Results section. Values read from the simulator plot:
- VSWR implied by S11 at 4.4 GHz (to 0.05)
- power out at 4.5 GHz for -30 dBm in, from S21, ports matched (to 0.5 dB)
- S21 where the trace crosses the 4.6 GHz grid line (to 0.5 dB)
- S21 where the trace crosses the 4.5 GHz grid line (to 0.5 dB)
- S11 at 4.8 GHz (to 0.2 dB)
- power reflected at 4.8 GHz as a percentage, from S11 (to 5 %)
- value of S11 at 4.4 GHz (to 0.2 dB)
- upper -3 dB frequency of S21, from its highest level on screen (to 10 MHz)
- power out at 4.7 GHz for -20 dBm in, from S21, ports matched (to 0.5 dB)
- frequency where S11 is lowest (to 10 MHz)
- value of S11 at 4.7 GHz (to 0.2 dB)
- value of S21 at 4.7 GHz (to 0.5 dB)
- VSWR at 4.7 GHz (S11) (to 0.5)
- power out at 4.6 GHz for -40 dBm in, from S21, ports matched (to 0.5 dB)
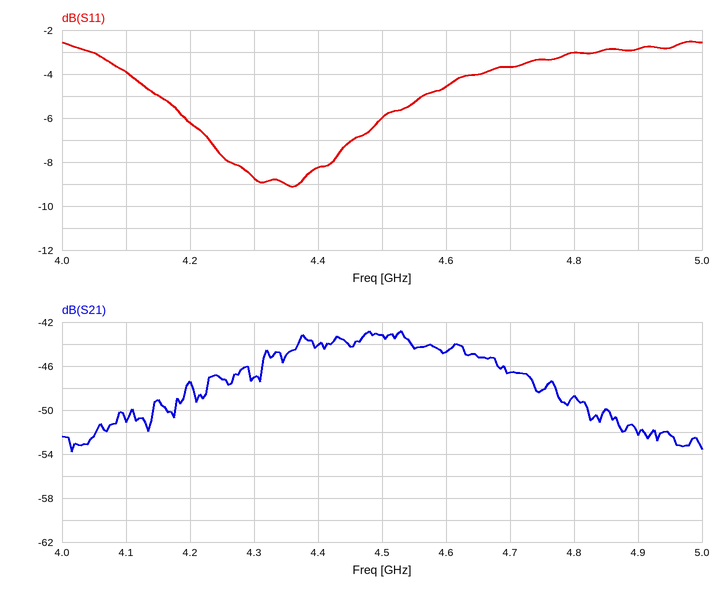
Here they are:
2.25
-73.0 dBm
-44.5 dB
-43.0 dB
-3.0 dB
50 %
-8.2 dB
4.68 GHz
-66.5 dBm
4.36 GHz
-3.6 dB
-46.5 dB
5.0
-84.5 dBm
